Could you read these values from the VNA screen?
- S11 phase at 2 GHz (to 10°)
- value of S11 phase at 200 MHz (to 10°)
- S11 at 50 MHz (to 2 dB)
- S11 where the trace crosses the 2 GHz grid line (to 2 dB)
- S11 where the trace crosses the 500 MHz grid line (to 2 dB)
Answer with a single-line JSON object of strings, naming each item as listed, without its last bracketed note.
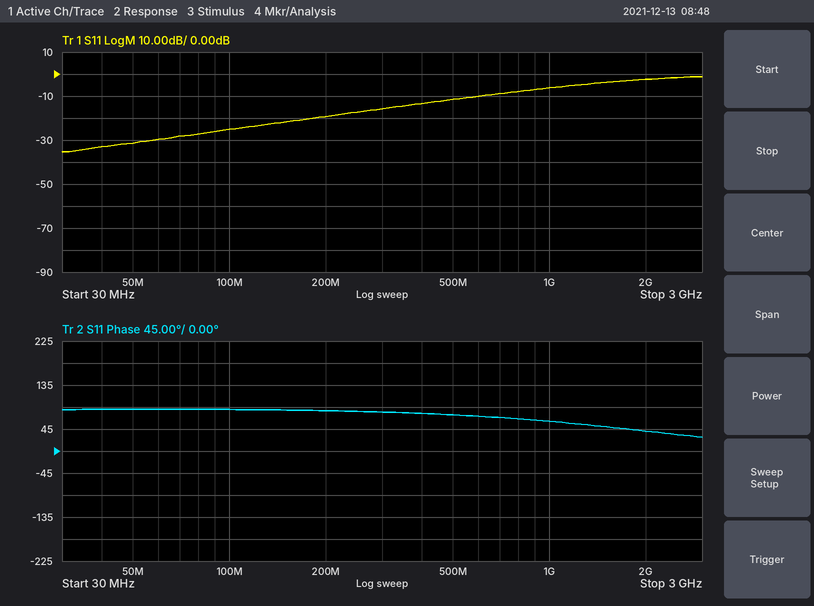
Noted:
{"S11 phase at 2 GHz": "40°", "value of S11 phase at 200 MHz": "80°", "S11 at 50 MHz": "-32 dB", "S11 where the trace crosses the 2 GHz grid line": "-2 dB", "S11 where the trace crosses the 500 MHz grid line": "-12 dB"}
